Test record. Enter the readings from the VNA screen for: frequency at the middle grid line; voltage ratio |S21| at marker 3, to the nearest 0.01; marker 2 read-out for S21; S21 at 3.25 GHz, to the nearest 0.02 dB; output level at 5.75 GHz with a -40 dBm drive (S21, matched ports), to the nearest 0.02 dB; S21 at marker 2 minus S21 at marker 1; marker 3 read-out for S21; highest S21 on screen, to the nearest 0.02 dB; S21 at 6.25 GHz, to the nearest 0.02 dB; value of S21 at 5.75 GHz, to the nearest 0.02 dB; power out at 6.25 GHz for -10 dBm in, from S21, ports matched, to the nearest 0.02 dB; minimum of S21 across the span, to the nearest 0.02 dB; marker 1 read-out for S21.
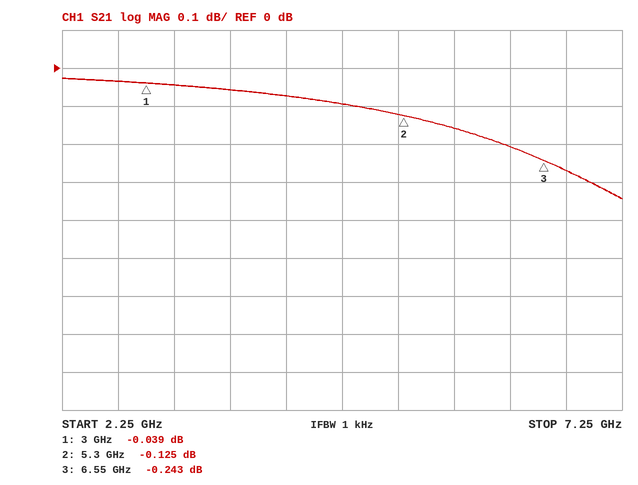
4.75 GHz
0.97
-0.125 dB
-0.04 dB
-40.16 dBm
-0.086 dB
-0.243 dB
-0.02 dB
-0.20 dB
-0.16 dB
-10.20 dBm
-0.34 dB
-0.039 dB
